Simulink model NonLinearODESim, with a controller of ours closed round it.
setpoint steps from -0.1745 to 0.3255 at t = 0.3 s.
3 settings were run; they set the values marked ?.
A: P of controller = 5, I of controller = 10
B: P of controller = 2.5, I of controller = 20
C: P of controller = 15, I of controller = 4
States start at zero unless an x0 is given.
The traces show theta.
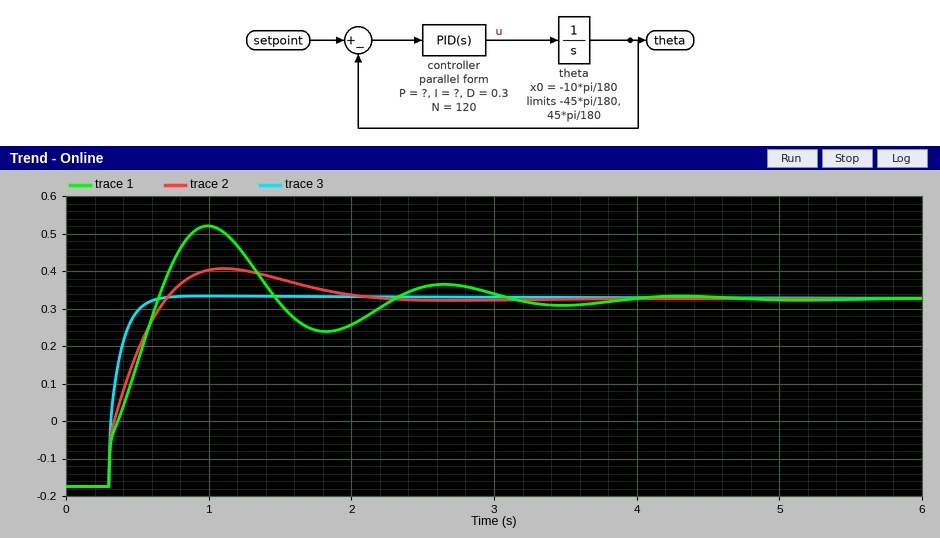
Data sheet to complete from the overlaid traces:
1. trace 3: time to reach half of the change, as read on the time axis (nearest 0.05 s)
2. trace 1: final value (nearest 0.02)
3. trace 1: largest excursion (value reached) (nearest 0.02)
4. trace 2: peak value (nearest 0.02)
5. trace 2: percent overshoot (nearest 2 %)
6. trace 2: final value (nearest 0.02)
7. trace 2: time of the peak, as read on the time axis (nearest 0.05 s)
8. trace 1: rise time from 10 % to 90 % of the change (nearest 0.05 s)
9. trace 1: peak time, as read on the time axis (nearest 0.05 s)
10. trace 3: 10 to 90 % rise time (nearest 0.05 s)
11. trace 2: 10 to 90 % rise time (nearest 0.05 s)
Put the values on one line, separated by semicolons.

0.35 s; 0.32; 0.52; 0.40; 16 %; 0.32; 1.10 s; 0.30 s; 1.00 s; 0.15 s; 0.30 s
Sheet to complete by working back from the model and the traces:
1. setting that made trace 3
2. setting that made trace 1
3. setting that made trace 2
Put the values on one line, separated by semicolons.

C; B; A
